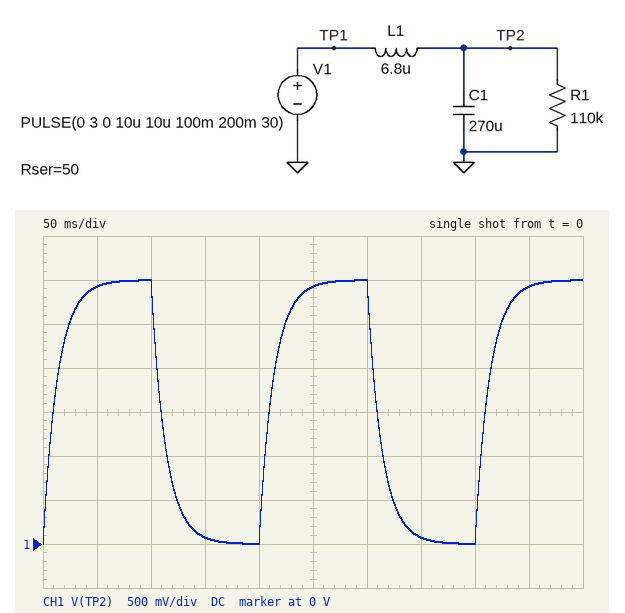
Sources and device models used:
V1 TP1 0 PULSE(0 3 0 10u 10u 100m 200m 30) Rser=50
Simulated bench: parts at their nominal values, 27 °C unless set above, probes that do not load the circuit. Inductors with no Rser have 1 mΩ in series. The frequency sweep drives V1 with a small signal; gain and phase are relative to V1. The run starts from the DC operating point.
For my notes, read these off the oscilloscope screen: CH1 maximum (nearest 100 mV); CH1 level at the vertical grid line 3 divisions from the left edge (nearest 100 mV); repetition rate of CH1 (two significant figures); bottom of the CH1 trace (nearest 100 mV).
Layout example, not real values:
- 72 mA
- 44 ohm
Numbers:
- 3.0 V
- 100 mV
- 5.0 Hz
- 0 V
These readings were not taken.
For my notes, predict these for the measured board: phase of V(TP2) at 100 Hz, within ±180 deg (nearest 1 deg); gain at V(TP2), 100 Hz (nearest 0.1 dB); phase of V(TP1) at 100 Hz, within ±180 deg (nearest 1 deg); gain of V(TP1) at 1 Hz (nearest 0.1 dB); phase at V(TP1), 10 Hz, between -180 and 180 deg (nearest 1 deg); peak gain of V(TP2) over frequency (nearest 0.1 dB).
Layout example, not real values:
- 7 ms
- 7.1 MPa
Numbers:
- -83 deg
- -18.6 dB
- -83 deg
- 0 dB
- -40 deg
- 0 dB
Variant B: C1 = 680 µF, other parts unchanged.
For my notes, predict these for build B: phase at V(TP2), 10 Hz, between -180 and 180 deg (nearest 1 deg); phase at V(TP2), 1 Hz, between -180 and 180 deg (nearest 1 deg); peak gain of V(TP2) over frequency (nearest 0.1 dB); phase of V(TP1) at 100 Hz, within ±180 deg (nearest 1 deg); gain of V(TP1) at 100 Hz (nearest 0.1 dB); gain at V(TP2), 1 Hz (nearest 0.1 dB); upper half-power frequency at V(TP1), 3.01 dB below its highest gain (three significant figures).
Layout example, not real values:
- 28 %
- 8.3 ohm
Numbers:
- -65 deg
- -12 deg
- 0 dB
- -87 deg
- -26.6 dB
- -0.2 dB
- 4.68 Hz
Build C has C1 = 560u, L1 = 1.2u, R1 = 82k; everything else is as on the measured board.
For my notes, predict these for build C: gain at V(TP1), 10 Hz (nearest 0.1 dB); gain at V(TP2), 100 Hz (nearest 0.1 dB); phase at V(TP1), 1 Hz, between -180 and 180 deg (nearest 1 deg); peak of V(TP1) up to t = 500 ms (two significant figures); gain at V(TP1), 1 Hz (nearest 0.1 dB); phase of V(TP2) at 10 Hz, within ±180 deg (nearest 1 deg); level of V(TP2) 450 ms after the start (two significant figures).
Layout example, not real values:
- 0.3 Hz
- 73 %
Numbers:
- -6.1 dB
- -24.9 dB
- -10 deg
- 2.9 V
- -0.1 dB
- -60 deg
- 2.5 V
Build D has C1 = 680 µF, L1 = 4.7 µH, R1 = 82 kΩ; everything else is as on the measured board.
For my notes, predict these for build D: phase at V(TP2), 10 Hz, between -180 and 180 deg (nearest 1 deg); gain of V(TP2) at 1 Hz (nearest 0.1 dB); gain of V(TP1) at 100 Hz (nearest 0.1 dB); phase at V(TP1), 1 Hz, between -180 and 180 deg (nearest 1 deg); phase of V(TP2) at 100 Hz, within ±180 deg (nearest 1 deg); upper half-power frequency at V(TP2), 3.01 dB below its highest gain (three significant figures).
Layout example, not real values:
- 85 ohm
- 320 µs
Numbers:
- -65 deg
- -0.2 dB
- -26.6 dB
- -12 deg
- -87 deg
- 4.68 Hz
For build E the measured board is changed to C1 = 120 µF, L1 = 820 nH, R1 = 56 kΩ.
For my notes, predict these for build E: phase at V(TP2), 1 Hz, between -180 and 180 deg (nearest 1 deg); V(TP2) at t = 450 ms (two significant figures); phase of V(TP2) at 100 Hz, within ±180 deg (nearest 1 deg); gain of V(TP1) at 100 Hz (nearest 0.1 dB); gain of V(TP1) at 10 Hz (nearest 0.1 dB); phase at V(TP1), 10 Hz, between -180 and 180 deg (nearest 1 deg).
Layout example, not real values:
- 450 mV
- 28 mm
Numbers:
- -2 deg
- 3.0 V
- -75 deg
- -11.8 dB
- -0.6 dB
- -21 deg
